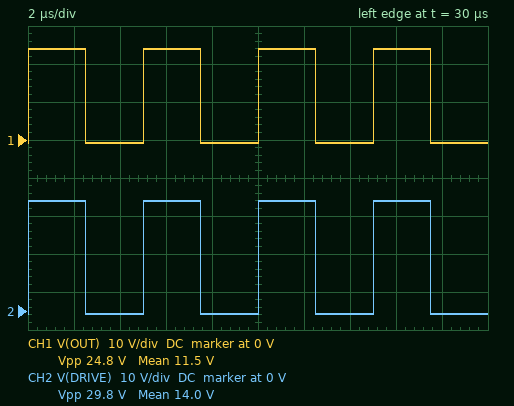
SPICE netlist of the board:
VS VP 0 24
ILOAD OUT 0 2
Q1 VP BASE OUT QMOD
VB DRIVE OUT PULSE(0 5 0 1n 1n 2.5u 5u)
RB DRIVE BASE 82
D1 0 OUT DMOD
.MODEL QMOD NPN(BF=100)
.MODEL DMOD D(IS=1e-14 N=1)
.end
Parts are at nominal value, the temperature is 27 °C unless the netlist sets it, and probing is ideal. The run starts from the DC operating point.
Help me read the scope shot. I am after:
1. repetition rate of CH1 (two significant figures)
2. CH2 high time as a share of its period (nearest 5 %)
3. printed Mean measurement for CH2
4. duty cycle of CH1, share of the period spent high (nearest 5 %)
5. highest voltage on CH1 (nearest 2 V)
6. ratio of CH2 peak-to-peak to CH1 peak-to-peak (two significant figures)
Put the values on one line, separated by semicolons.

200 kHz; 50 %; 14.0 V; 50 %; 24 V; 1.2
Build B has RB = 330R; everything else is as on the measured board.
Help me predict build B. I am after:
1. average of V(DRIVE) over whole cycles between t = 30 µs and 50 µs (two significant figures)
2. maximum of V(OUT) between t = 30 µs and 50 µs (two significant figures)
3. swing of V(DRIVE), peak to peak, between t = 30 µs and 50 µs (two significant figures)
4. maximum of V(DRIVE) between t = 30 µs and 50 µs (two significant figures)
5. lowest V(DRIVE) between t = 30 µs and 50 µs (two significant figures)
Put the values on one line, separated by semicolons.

1.7 V; -830 mV; 5.0 V; 4.2 V; -850 mV
